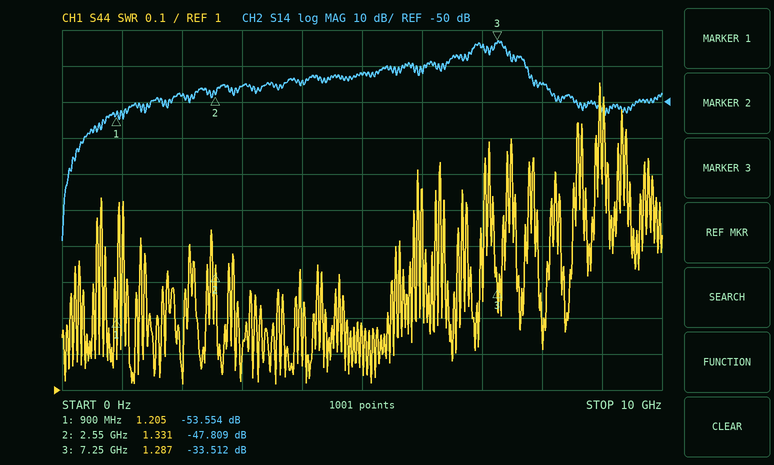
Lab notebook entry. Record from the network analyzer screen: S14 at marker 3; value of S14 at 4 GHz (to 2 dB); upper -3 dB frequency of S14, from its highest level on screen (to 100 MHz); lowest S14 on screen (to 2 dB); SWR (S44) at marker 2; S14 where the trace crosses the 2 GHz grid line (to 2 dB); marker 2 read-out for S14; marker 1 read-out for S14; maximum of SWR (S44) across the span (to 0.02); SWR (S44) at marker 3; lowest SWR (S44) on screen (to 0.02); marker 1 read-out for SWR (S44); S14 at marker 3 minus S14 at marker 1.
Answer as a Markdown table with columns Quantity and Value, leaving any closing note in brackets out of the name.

| Quantity | Value |
|---|---|
| S14 at marker 3 | -33.512 dB |
| value of S14 at 4 GHz | -44 dB |
| upper -3 dB frequency of S14, from its highest level on screen | 7.4 GHz |
| lowest S14 on screen | -88 dB |
| SWR (S44) at marker 2 | 1.331 |
| S14 where the trace crosses the 2 GHz grid line | -48 dB |
| marker 2 read-out for S14 | -47.809 dB |
| marker 1 read-out for S14 | -53.554 dB |
| maximum of SWR (S44) across the span | 1.86 |
| SWR (S44) at marker 3 | 1.287 |
| lowest SWR (S44) on screen | 1.02 |
| marker 1 read-out for SWR | 1.205 |
| S14 at marker 3 minus S14 at marker 1 | 20.042 dB |
